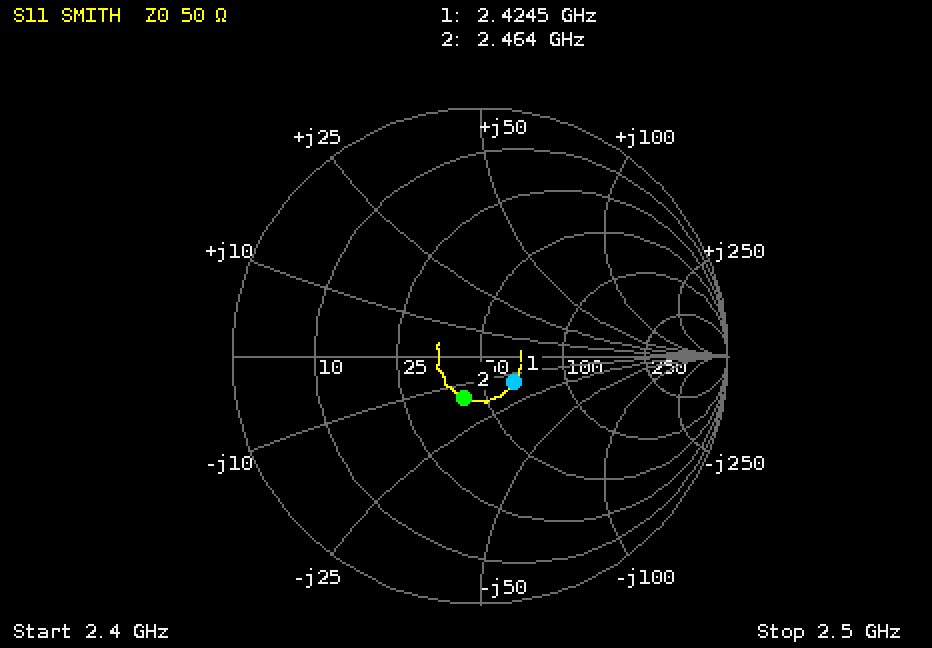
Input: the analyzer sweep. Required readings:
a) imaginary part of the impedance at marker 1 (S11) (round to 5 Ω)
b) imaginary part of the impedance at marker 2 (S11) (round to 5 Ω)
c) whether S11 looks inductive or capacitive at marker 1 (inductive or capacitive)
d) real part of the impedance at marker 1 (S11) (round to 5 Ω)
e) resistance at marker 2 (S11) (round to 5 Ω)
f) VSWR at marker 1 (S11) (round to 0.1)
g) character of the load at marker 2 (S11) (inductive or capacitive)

-15 Ω
-15 Ω
capacitive
65 Ω
40 Ω
1.4
capacitive
